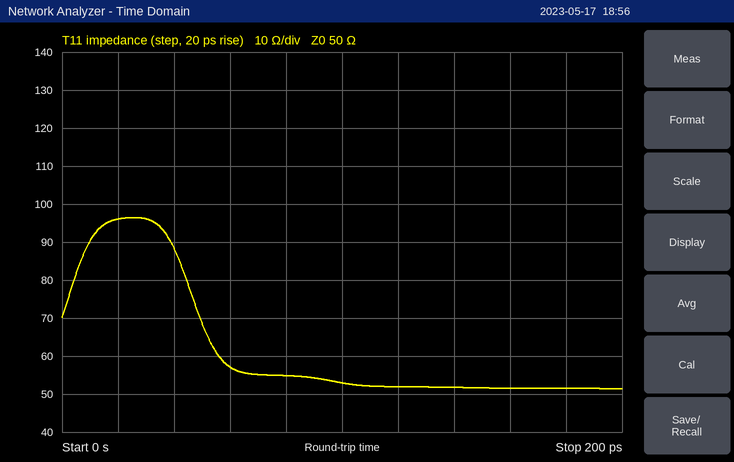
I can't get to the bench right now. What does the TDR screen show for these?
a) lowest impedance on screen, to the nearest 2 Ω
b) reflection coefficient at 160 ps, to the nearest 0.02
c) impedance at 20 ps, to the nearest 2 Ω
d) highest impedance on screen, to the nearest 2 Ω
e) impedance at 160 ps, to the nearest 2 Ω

52 Ω
+0.02
96 Ω
96 Ω
52 Ω
